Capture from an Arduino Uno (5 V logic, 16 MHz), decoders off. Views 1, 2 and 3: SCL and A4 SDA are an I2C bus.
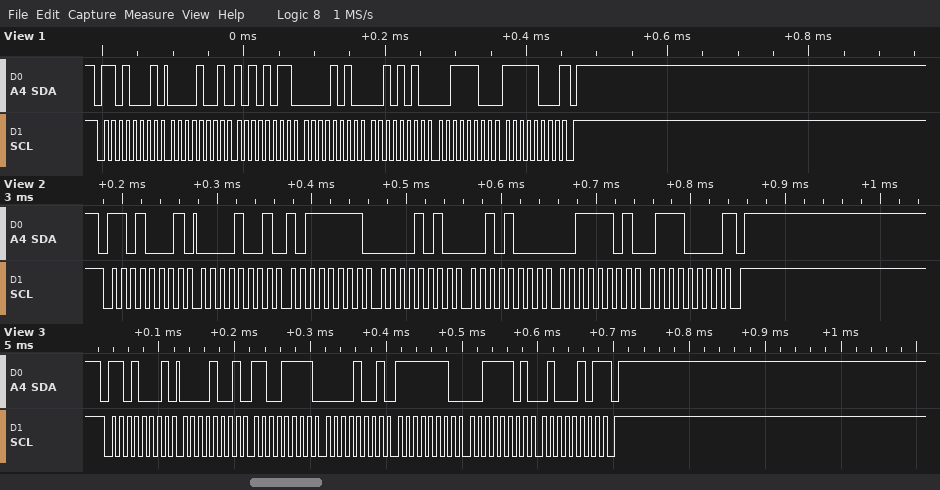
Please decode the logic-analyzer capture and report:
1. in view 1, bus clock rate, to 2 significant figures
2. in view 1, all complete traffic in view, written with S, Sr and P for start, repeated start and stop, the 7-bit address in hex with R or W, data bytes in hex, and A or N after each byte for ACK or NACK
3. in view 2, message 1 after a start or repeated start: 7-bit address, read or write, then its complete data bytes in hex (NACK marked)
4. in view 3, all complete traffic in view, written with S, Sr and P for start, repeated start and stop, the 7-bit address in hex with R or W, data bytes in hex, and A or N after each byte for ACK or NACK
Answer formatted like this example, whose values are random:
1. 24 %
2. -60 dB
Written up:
1. 100 kHz
2. S 68R A 09 A AB A 0A A 2A A 3C A F8 N P
3. 0x68 read: 09 BF 0A 28 3D 70 NACK
4. S 68R A 09 A CF A 09 A FE A 3D A 45 N P
